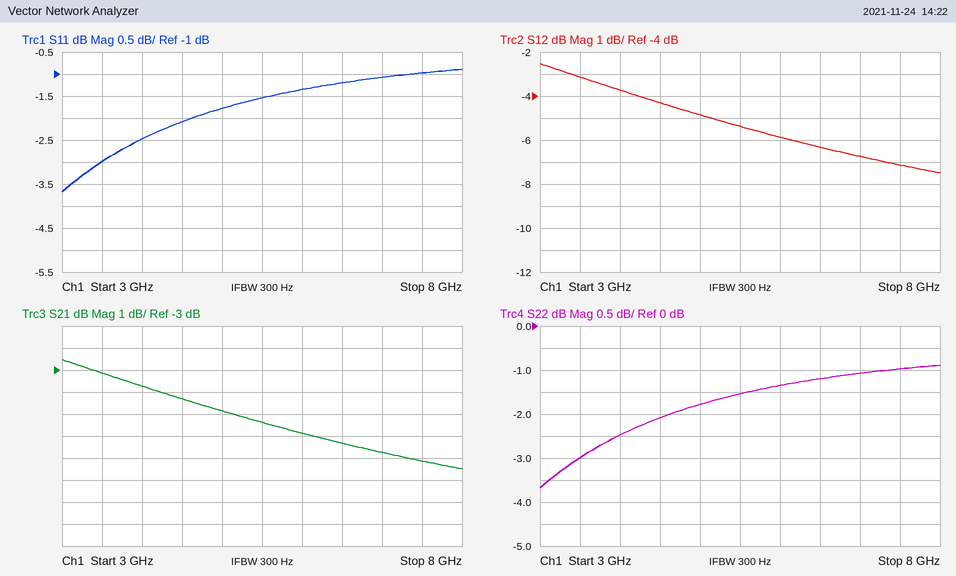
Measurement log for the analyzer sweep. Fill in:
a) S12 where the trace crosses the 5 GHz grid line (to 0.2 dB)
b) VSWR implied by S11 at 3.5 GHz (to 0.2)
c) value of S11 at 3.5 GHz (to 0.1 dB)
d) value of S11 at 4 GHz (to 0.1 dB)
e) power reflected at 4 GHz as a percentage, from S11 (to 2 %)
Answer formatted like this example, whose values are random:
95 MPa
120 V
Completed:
-4.8 dB
5.8
-3.0 dB
-2.5 dB
56 %
